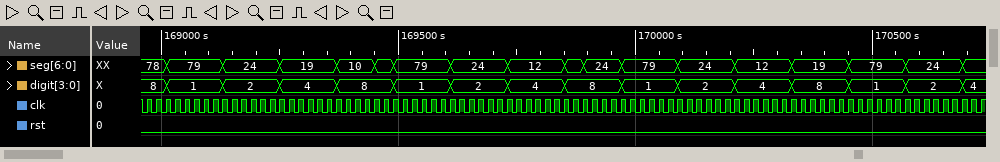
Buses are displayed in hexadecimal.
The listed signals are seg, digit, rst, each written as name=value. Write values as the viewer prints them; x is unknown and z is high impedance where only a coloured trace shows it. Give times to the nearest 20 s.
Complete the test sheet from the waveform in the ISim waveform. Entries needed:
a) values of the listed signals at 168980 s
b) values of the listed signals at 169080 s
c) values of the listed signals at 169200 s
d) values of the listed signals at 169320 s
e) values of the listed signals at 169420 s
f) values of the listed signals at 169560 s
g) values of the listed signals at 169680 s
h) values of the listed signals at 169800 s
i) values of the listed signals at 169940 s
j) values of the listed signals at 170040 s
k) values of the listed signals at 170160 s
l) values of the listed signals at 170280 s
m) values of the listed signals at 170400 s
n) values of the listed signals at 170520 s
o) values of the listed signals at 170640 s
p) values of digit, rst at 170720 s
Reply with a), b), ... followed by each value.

a) seg=78, digit=8, rst=0
b) seg=79, digit=1, rst=0
c) seg=24, digit=2, rst=0
d) seg=19, digit=4, rst=0
e) seg=10, digit=8, rst=0
f) seg=79, digit=1, rst=0
g) seg=24, digit=2, rst=0
h) seg=12, digit=4, rst=0
i) seg=24, digit=8, rst=0
j) seg=79, digit=1, rst=0
k) seg=24, digit=2, rst=0
l) seg=12, digit=4, rst=0
m) seg=19, digit=8, rst=0
n) seg=79, digit=1, rst=0
o) seg=24, digit=2, rst=0
p) digit=4, rst=0
